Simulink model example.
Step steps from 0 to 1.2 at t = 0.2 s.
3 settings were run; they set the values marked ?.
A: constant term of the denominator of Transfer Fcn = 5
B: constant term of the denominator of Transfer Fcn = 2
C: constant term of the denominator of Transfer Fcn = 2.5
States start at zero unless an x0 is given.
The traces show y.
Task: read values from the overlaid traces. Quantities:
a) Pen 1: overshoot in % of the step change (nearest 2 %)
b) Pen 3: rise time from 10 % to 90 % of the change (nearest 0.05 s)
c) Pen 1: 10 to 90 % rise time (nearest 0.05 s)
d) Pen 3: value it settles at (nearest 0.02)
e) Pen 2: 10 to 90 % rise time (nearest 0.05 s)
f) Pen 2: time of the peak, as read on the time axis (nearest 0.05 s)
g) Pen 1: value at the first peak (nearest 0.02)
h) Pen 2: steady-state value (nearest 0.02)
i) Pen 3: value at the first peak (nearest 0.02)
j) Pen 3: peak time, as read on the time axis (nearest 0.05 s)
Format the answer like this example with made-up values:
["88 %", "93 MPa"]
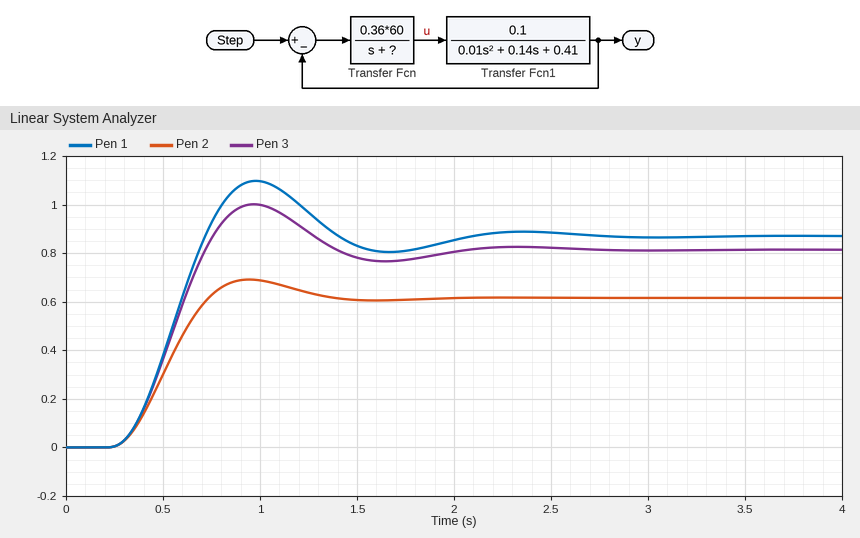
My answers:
["26 %", "0.30 s", "0.30 s", "0.82", "0.35 s", "0.95 s", "1.10", "0.62", "1.00", "0.95 s"]
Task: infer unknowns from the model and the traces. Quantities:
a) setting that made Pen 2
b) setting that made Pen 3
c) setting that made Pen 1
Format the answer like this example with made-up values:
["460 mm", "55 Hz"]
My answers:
["A", "C", "B"]
